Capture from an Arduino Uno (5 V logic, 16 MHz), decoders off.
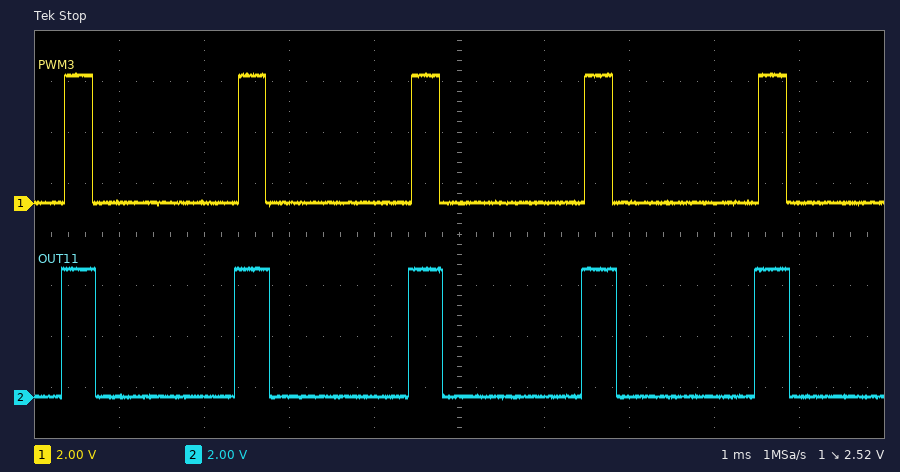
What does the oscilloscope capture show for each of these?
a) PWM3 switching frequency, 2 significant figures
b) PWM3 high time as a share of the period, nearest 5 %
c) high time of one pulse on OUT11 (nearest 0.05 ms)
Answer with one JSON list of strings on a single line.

["490 Hz", "15 %", "0.40 ms"]
